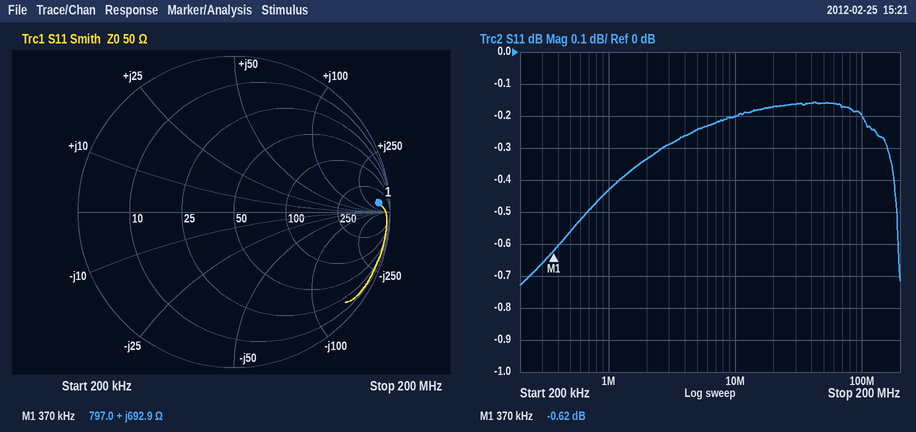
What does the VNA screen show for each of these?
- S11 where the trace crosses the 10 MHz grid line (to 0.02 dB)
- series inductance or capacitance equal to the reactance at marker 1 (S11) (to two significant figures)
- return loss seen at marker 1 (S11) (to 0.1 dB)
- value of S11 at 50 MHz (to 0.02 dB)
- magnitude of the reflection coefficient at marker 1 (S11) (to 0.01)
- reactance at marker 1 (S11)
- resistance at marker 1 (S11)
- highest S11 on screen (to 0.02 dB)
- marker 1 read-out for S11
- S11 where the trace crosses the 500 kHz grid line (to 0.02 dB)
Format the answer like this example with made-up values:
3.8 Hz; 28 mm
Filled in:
-0.20 dB; 300 µH; 0.6 dB; -0.16 dB; 0.93; +692.9 Ω; 797.0 Ω; -0.16 dB; -0.62 dB; -0.56 dB
